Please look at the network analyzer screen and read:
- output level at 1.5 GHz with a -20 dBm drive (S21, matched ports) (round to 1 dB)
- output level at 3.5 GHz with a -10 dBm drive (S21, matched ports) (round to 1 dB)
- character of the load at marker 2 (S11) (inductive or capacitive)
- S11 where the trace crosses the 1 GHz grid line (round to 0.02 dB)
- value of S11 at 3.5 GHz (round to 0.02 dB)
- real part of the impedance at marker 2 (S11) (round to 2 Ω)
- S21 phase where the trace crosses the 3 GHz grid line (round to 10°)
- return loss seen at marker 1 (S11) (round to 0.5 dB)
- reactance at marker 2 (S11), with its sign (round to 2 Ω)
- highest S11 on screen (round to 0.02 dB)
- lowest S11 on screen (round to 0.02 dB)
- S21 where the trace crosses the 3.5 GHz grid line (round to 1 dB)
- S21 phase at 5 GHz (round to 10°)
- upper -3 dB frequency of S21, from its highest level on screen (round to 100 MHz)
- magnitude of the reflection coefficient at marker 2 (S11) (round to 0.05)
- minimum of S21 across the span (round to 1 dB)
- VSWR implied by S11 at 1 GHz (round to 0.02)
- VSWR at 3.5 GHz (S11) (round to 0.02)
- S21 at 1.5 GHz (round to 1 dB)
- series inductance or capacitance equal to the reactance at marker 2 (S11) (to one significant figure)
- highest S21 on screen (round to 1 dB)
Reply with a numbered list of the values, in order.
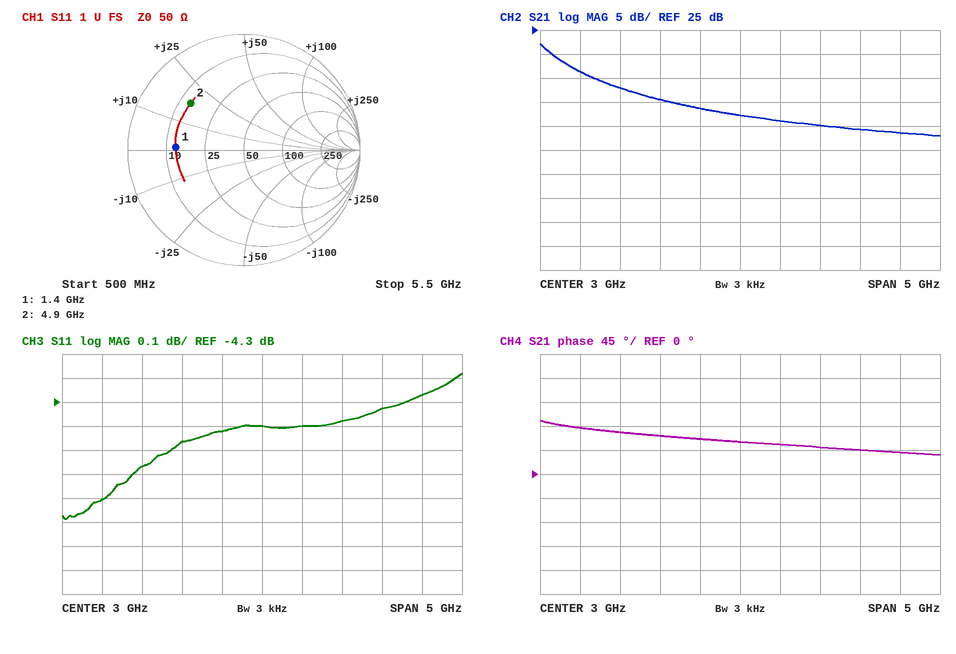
1. -7 dBm
2. -4 dBm
3. inductive
4. -4.70 dB
5. -4.40 dB
6. 14 Ω
7. 60°
8. 4.5 dB
9. +18 Ω
10. -4.18 dB
11. -4.78 dB
12. 6 dB
13. 40°
14. 700 MHz
15. 0.60
16. 3 dB
17. 3.78
18. 4.04
19. 13 dB
20. 600 pH
21. 22 dB
